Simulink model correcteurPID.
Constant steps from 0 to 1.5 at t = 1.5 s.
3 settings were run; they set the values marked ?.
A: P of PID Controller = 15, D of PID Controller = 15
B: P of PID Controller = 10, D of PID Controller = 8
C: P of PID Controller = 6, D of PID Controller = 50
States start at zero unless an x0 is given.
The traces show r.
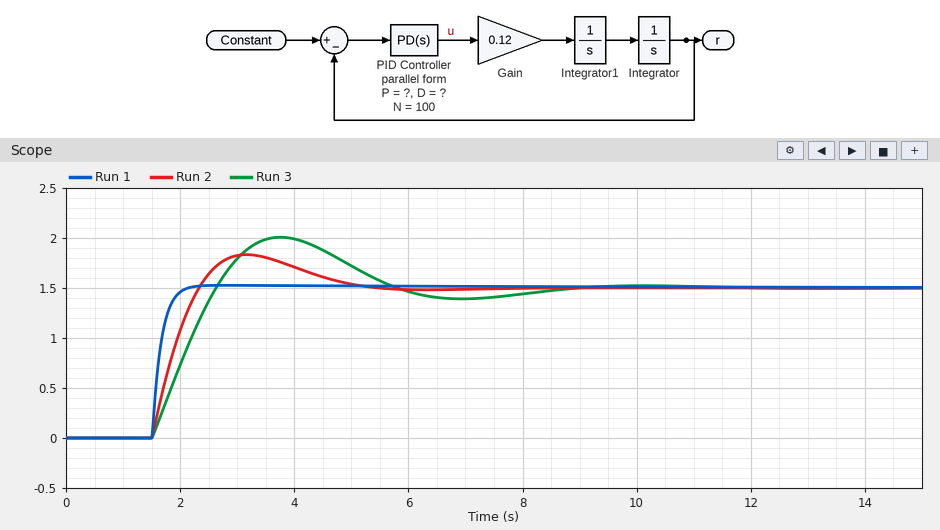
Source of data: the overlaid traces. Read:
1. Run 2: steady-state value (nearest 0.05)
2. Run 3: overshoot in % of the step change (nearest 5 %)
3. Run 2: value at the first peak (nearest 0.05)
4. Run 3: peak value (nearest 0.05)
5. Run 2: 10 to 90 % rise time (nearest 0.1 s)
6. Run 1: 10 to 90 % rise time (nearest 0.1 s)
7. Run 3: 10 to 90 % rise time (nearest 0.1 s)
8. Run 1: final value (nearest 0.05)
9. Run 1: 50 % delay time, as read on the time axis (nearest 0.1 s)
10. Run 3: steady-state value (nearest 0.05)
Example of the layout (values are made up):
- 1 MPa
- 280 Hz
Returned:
- 1.50
- 35 %
- 1.85
- 2.00
- 0.6 s
- 0.3 s
- 0.9 s
- 1.50
- 1.6 s
- 1.50
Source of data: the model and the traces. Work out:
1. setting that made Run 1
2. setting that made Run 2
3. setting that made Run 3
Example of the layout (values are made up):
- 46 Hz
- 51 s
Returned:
- C
- A
- B
